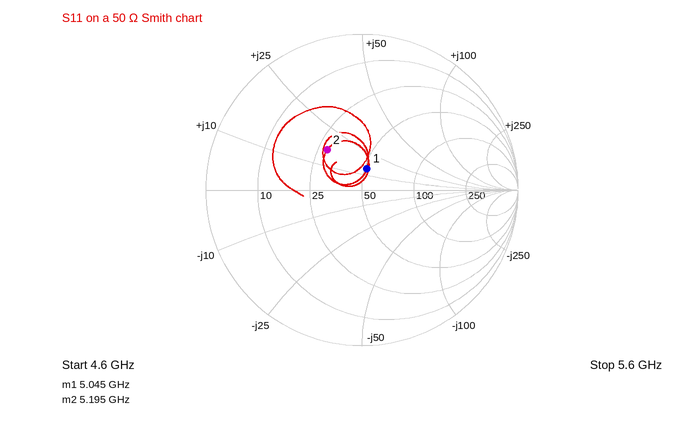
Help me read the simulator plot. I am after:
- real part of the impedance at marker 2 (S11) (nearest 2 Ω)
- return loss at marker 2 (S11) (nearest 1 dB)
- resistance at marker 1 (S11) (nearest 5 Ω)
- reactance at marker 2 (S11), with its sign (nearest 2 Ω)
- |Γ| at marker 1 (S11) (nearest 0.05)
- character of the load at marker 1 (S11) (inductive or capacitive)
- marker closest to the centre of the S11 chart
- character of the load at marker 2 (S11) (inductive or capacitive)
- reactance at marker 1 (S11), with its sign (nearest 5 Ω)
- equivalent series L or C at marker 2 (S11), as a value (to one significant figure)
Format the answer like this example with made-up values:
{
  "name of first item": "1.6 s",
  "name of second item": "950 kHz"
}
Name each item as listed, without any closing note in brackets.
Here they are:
{
  "real part of the impedance at marker 2 (S11)": "28 Ω",
  "return loss at marker 2 (S11)": "9 dB",
  "resistance at marker 1 (S11)": "50 Ω",
  "reactance at marker 2 (S11), with its sign": "+16 Ω",
  "|Γ| at marker 1 (S11)": "0.15",
  "character of the load at marker 1 (S11)": "inductive",
  "marker closest to the centre of the S11 chart": "marker 1",
  "character of the load at marker 2 (S11)": "inductive",
  "reactance at marker 1 (S11), with its sign": "+15 Ω",
  "equivalent series L or C at marker 2 (S11), as a value": "500 pH"
}
